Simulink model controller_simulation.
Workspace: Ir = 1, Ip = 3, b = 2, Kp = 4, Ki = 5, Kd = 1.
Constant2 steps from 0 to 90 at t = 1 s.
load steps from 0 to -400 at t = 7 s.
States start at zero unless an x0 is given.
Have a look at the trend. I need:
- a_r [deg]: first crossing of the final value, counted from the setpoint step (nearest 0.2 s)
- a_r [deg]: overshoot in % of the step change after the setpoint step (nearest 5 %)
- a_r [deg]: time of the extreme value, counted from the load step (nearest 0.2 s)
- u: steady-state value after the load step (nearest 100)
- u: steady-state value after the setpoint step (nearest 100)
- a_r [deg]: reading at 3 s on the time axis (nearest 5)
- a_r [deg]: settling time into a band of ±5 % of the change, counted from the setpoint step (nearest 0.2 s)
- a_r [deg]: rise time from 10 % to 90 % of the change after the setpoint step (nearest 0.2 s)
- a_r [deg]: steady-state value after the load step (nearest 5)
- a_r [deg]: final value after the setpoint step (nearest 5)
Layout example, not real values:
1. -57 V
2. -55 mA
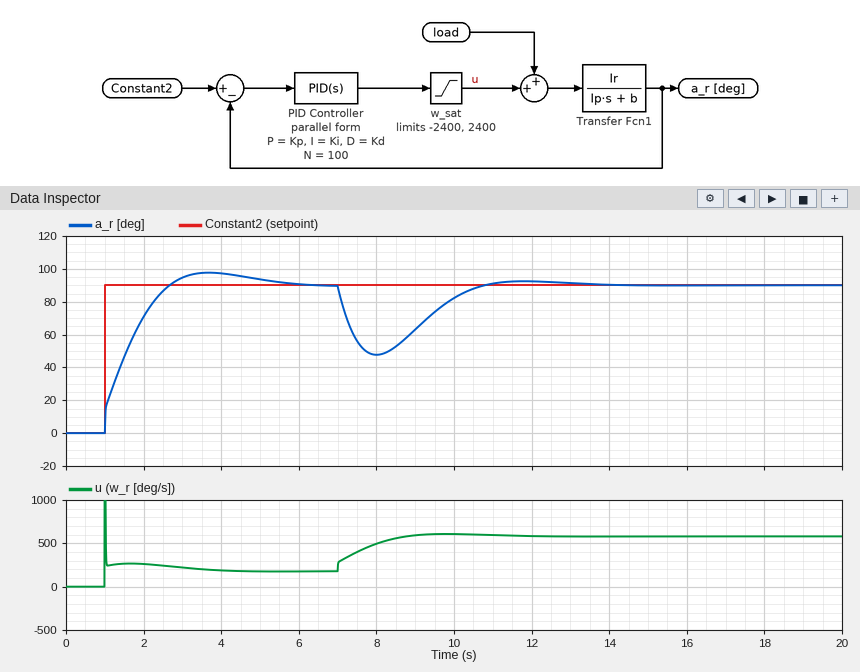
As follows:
1. 1.6 s
2. 10 %
3. 1.0 s
4. 600
5. 200
6. 95
7. 3.8 s
8. 1.2 s
9. 90
10. 90
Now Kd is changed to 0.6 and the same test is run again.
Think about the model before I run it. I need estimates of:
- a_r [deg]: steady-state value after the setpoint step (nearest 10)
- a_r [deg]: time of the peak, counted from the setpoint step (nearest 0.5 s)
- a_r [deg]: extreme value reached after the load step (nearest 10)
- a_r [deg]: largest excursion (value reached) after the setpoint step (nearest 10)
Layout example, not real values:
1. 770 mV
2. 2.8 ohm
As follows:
1. 90
2. 2.5 s
3. 50
4. 100
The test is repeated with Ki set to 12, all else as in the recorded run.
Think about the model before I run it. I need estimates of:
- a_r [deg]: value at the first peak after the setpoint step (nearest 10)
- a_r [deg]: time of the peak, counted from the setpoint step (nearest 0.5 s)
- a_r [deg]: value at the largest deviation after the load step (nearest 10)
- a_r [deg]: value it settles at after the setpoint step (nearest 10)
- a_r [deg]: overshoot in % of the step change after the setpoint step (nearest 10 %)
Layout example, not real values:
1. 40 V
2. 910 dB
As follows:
1. 110
2. 1.5 s
3. 60
4. 90
5. 20 %
